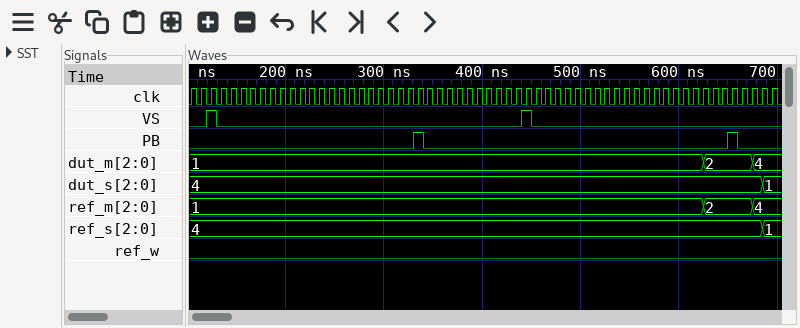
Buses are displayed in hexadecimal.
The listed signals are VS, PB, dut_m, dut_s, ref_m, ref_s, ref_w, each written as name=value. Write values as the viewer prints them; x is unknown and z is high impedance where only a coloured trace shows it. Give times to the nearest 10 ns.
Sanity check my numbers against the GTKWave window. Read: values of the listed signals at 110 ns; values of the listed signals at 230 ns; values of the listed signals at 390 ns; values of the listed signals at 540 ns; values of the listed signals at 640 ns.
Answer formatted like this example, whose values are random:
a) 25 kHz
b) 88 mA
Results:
a) VS=0, PB=0, dut_m=1, dut_s=4, ref_m=1, ref_s=4, ref_w=0
b) VS=0, PB=0, dut_m=1, dut_s=4, ref_m=1, ref_s=4, ref_w=0
c) VS=0, PB=0, dut_m=1, dut_s=4, ref_m=1, ref_s=4, ref_w=0
d) VS=0, PB=0, dut_m=1, dut_s=4, ref_m=1, ref_s=4, ref_w=0
e) VS=0, PB=0, dut_m=2, dut_s=4, ref_m=2, ref_s=4, ref_w=0
